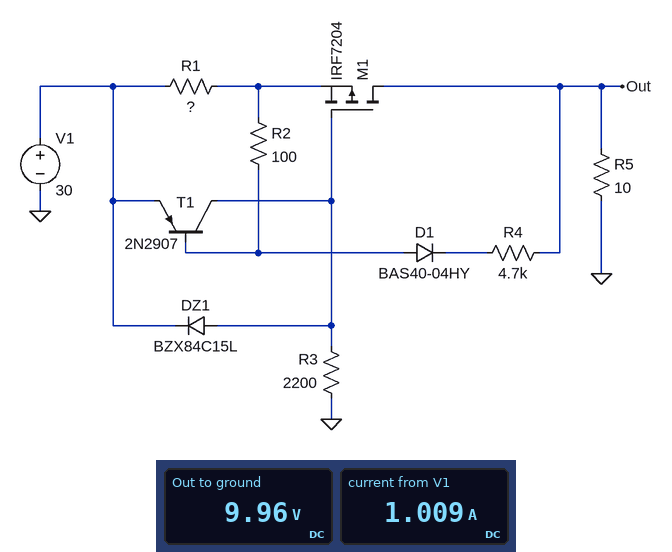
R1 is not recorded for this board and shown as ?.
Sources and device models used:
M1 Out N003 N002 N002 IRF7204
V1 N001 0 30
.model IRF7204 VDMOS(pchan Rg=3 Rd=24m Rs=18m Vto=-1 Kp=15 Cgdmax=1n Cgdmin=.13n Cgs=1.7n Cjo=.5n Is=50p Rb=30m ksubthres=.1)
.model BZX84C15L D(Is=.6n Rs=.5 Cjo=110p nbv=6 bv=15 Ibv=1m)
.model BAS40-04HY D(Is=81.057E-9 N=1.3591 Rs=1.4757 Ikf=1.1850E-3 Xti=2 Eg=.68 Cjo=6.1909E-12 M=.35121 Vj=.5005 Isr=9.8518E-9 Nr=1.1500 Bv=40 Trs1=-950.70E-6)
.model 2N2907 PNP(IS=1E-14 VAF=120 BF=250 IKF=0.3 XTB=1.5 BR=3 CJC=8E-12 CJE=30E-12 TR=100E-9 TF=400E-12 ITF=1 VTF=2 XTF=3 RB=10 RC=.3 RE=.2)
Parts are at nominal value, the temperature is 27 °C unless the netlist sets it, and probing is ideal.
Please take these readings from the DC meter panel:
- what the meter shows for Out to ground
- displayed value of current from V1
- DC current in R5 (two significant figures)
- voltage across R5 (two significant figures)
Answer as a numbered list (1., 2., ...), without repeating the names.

1. 9.96 V
2. 1.009 A
3. 1.0 A
4. 10 V
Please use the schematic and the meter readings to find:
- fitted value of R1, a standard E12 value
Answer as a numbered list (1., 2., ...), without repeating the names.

1. 0.33 Ω
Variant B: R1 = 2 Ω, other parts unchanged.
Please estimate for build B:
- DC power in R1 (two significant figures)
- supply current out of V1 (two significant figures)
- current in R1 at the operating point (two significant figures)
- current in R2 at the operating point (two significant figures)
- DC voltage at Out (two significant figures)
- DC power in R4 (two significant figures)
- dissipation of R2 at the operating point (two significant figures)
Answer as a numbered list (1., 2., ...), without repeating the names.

1. 8.7 mW
2. 79 mA
3. 66 mA
4. 5.9 mA
5. 660 mV
6. 170 mW
7. 3.5 mW
